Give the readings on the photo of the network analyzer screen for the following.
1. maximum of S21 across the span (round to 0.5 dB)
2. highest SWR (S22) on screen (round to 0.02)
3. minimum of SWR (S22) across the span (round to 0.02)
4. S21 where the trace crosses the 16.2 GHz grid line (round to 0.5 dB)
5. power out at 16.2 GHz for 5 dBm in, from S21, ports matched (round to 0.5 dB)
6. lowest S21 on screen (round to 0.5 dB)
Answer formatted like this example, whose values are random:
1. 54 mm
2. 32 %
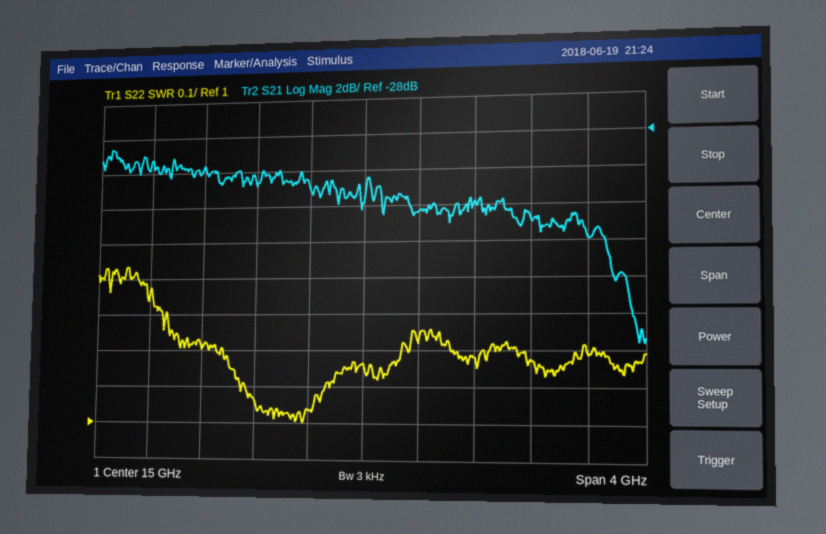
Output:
1. -28.5 dB
2. 1.44
3. 1.00
4. -33.0 dB
5. -28.0 dBm
6. -39.5 dB
